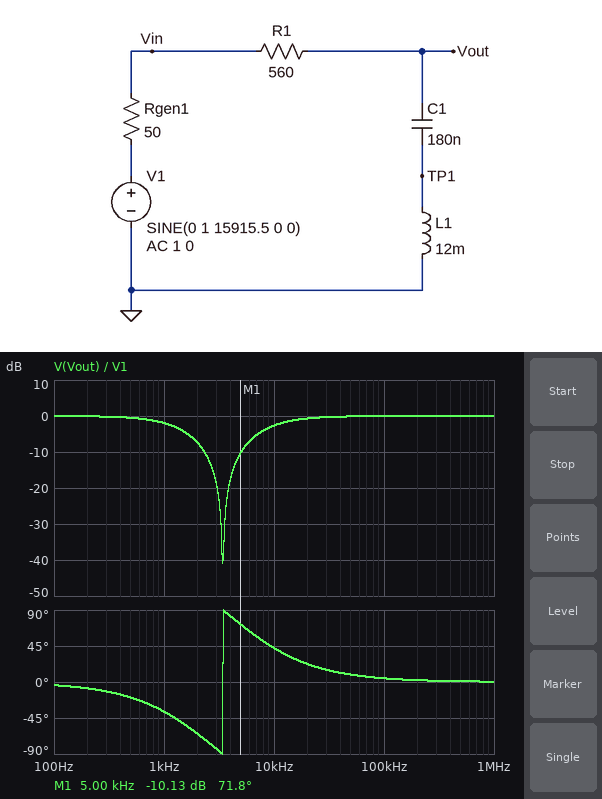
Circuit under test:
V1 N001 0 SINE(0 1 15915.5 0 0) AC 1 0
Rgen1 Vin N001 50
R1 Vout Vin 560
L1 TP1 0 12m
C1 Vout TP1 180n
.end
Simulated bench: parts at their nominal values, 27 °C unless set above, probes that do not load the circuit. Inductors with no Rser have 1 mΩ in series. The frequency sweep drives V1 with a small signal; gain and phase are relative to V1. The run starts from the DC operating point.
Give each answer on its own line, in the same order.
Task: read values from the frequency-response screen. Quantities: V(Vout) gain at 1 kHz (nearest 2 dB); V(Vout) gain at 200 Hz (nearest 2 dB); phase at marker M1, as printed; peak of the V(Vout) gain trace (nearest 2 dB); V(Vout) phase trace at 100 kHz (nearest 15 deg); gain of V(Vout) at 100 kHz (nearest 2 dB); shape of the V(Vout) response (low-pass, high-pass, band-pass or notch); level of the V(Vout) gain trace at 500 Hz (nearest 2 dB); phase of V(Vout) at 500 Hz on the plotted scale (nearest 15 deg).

-2 dB
0 dB
71.8 deg
0 dB
0 deg
0 dB
notch
0 dB
-15 deg
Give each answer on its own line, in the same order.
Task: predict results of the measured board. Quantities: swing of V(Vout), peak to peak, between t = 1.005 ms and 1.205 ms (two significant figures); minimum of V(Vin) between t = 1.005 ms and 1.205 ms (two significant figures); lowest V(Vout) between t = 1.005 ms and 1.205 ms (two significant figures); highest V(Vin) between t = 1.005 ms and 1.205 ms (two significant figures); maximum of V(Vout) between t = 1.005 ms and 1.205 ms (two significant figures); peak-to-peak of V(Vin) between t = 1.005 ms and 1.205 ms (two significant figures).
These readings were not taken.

1.8 V
-980 mV
-880 mV
980 mV
880 mV
2.0 V
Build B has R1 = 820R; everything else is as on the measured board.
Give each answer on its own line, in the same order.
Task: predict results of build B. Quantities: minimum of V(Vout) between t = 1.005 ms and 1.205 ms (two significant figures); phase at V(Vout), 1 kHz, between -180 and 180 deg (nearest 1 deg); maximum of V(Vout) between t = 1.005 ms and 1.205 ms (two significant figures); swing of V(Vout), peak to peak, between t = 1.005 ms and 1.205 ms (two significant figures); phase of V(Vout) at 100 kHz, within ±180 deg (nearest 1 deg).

-800 mV
-47 deg
800 mV
1.6 V
7 deg
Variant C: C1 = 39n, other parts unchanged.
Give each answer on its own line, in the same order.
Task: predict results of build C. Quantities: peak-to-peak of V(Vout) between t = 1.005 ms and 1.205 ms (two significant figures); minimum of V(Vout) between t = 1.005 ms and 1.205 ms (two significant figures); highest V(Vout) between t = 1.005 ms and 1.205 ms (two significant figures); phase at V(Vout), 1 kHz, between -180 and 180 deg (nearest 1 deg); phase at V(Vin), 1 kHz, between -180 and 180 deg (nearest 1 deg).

1.7 V
-840 mV
840 mV
-9 deg
-1 deg
